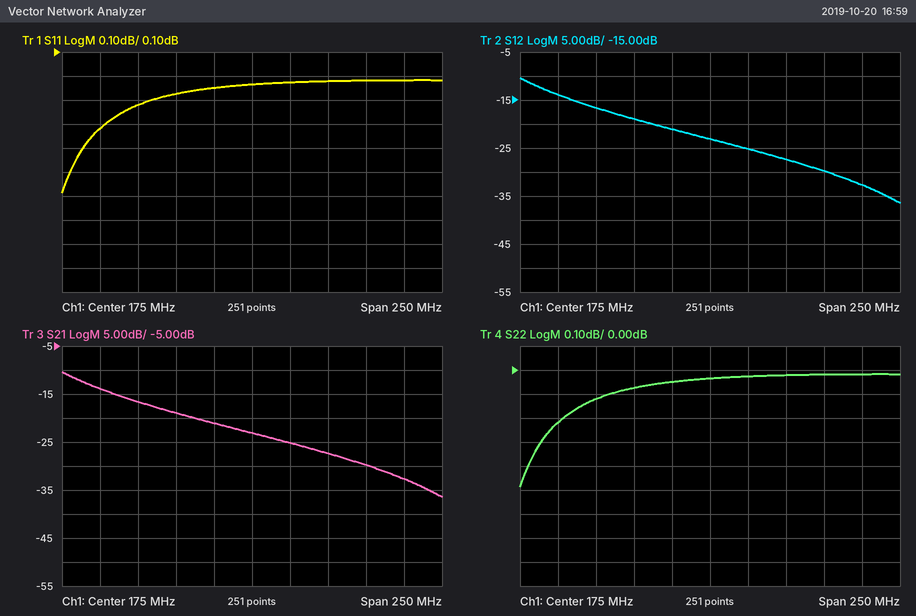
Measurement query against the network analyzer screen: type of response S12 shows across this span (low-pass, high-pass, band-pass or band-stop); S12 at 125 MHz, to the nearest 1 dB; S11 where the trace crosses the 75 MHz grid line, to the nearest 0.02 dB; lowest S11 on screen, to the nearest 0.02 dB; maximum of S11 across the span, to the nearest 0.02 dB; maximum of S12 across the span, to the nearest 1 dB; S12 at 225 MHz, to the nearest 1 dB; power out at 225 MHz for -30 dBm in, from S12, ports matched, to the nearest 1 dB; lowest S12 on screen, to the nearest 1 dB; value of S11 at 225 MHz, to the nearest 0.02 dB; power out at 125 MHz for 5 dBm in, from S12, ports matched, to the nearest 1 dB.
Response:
low-pass
-19 dB
-0.22 dB
-0.48 dB
-0.02 dB
-10 dB
-27 dB
-57 dBm
-36 dB
-0.02 dB
-14 dBm
